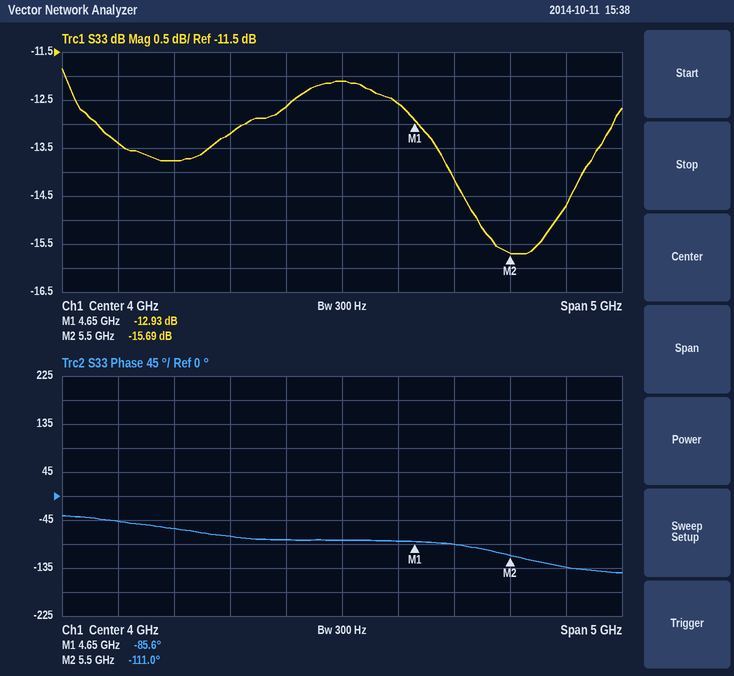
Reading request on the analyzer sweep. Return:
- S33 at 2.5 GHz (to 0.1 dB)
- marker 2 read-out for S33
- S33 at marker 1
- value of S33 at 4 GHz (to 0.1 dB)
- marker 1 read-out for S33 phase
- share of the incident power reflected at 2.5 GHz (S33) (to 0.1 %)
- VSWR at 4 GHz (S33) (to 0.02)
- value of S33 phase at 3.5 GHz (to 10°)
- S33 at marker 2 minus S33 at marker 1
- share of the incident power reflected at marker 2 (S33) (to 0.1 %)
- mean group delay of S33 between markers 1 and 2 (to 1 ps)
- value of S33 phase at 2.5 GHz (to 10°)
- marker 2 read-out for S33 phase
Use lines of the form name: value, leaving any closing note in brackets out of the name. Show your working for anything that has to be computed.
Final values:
S33 at 2.5 GHz: -13.8 dB
marker 2 read-out for S33: -15.69 dB
S33 at marker 1: -12.93 dB
value of S33 at 4 GHz: -12.1 dB
marker 1 read-out for S33 phase: -85.6°
share of the incident power reflected at 2.5 GHz (S33): 10^(-13.8/10) ≈ 4.2 %
VSWR at 4 GHz (S33): |Γ| = 10^(-12.1/20) = 0.2483; VSWR = (1 + 0.2483)/(1 − 0.2483) ≈ 1.66
value of S33 phase at 3.5 GHz: -80°
S33 at marker 2 minus S33 at marker 1: -15.69 − (-12.93) = -2.76 dB
share of the incident power reflected at marker 2 (S33): 10^(-15.69/10) ≈ 2.7 %
mean group delay of S33 between markers 1 and 2: −(-111° − (-85.6°))/(360° × 850 MHz) ≈ 83 ps
value of S33 phase at 2.5 GHz: -60°
marker 2 read-out for S33 phase: -111.0°
